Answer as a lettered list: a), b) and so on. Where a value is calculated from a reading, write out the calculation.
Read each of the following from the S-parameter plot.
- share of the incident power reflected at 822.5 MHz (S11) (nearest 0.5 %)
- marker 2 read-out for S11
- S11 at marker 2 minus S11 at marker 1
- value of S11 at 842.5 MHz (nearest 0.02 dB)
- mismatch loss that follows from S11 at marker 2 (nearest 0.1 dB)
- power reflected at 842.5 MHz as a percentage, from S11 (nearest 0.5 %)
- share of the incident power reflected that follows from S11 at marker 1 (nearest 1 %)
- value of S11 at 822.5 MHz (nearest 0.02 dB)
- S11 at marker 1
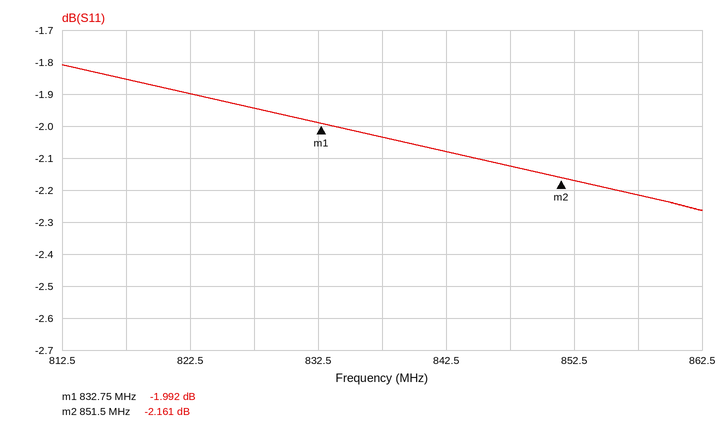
a) 10^(-1.9/10) ≈ 64.6 %, so 64.5 % to the nearest 0.5 %
b) -2.161 dB
c) -2.161 − (-1.992) = -0.169 dB
d) -2.08 dB
e) −10 log10(1 − 10^(-2.161/10)) ≈ 4.1 dB
f) 10^(-2.08/10) ≈ 61.9 %, so 62.0 % to the nearest 0.5 %
g) 10^(-1.992/10) ≈ 63 %
h) -1.90 dB
i) -1.992 dB
